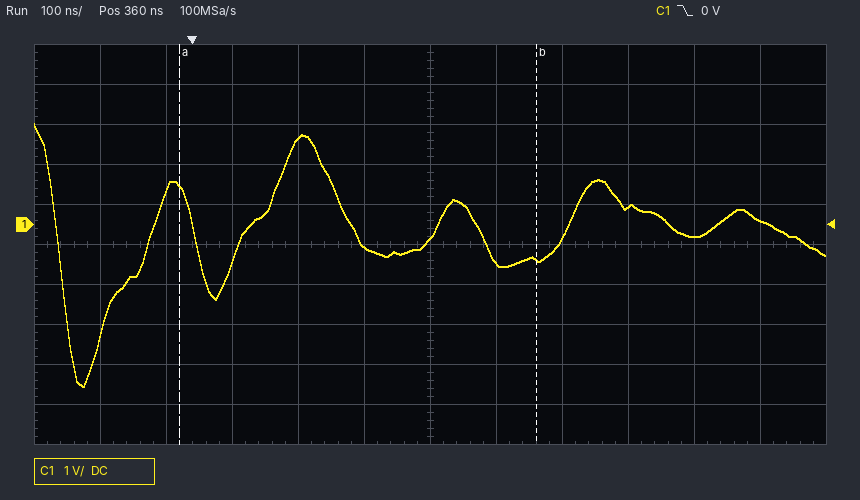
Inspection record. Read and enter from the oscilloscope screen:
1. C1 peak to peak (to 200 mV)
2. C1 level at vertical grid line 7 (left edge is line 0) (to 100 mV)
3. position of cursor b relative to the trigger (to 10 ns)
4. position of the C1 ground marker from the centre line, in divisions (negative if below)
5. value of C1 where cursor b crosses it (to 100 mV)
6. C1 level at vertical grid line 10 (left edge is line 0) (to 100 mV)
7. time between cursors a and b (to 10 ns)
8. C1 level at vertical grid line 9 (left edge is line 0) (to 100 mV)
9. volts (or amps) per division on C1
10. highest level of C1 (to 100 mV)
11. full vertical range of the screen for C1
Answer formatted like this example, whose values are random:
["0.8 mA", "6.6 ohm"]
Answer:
["6.6 V", "-1.0 V", "+520 ns", "+0.5 div", "-900 mV", "-300 mV", "540 ns", "400 mV", "1 V", "2.5 V", "10 V"]
